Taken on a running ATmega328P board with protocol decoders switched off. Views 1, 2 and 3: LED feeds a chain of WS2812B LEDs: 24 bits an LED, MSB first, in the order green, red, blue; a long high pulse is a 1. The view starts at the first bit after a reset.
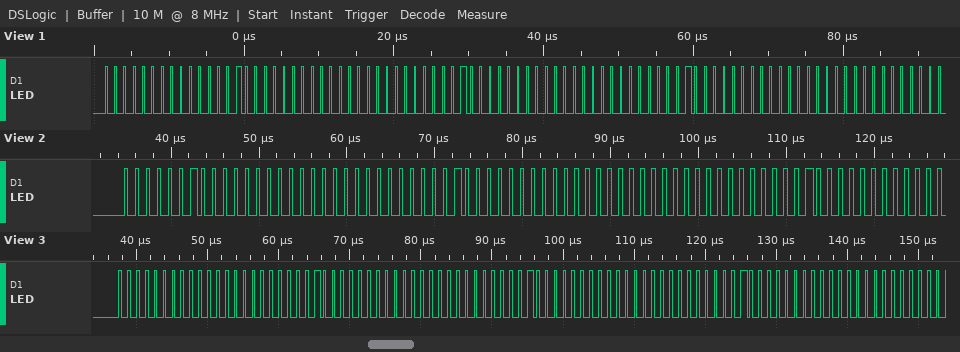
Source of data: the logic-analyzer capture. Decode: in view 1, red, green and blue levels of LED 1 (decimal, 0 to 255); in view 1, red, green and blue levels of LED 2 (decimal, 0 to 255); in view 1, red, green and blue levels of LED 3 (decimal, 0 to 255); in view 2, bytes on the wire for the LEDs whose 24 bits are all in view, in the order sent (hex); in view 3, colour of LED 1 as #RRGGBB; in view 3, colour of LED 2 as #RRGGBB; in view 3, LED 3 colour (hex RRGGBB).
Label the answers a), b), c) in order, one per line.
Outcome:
a) 2, 0, 0
b) 2, 0, 0
c) 2, 0, 0
d) 02 00 00 02 00 00 00 02 00
e) #000002
f) #000002
g) #000002
